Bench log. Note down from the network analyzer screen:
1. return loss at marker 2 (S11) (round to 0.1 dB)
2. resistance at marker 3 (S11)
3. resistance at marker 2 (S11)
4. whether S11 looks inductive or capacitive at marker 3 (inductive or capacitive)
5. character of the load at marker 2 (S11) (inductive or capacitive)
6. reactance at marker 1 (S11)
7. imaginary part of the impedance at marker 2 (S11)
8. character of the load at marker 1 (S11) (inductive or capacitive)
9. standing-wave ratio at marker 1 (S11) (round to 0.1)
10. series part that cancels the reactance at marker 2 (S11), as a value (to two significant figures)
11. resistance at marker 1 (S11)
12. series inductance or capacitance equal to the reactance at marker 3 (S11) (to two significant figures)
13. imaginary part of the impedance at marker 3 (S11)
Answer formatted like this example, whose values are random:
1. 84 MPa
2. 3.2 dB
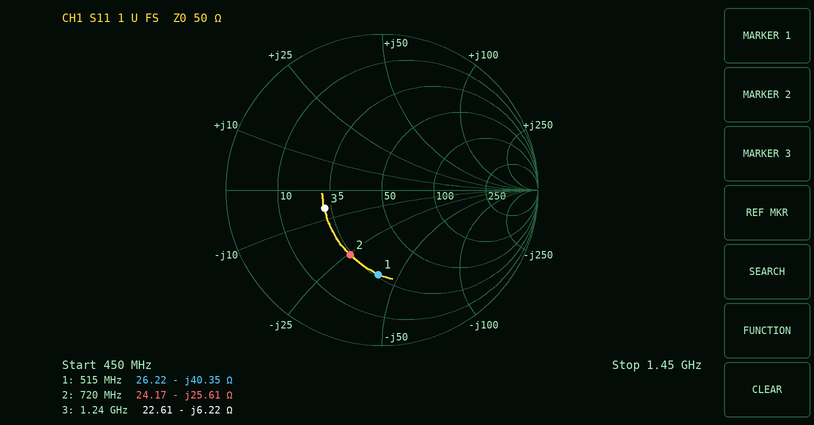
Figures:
1. 6.7 dB
2. 22.61 Ω
3. 24.17 Ω
4. capacitive
5. capacitive
6. -40.35 Ω
7. -25.61 Ω
8. capacitive
9. 3.4
10. 5.7 nH
11. 26.22 Ω
12. 21 pF
13. -6.22 Ω
